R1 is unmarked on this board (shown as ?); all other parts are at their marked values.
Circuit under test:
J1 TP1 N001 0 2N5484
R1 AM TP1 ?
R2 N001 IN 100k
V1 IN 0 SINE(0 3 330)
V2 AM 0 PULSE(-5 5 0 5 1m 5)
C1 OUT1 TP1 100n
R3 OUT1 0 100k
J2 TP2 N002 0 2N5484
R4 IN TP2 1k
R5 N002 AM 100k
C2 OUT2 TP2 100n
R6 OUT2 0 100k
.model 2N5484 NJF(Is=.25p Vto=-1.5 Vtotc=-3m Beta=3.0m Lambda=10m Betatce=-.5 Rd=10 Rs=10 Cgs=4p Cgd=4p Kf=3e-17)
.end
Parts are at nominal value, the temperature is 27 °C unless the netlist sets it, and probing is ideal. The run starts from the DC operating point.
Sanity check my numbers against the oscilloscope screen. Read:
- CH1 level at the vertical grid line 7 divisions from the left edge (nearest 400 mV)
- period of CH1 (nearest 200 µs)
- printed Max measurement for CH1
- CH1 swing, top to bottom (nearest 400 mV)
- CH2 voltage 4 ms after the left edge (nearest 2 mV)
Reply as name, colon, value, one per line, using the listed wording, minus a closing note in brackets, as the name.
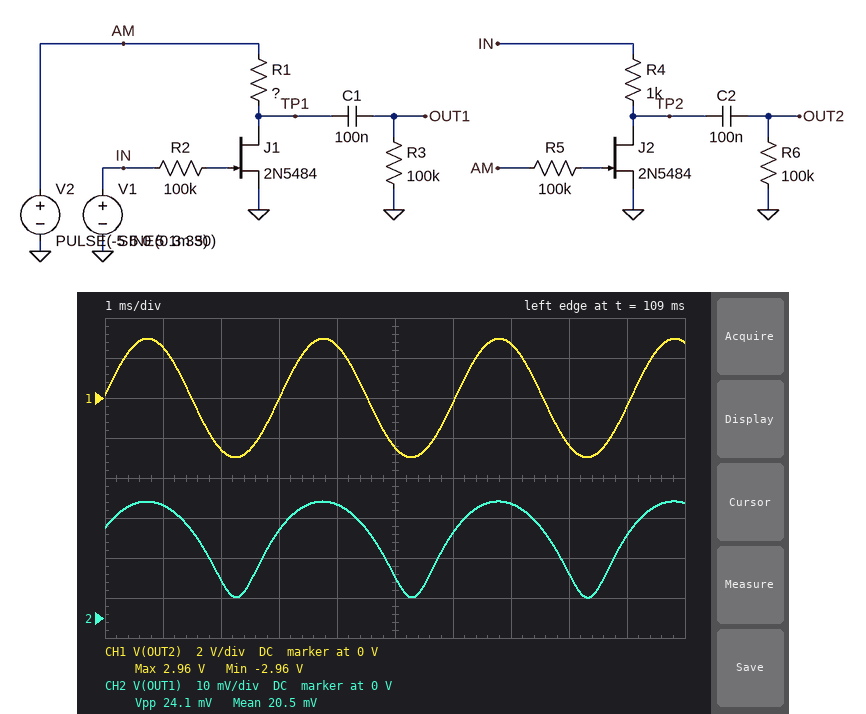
CH1 level at the vertical grid line 7 divisions from the left edge: 2.8 V
period of CH1: 3.0 ms
printed Max measurement for CH1: 2.96 V
CH1 swing, top to bottom: 6.0 V
CH2 voltage 4 ms after the left edge: 28 mV
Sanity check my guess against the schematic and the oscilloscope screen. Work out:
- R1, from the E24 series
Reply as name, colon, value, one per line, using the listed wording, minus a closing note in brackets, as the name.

R1, from the E24 series: 33 Ω
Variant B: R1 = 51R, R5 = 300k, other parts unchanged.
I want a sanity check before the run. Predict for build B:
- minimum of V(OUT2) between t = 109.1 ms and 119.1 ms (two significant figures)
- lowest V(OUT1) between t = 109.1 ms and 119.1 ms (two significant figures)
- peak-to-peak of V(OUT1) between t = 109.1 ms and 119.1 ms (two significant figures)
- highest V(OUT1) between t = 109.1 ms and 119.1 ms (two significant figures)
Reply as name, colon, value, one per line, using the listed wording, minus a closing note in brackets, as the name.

minimum of V(OUT2) between t = 109.1 ms and 119.1 ms: -3.0 V
lowest V(OUT1) between t = 109.1 ms and 119.1 ms: -5.9 mV
peak-to-peak of V(OUT1) between t = 109.1 ms and 119.1 ms: 41 mV
highest V(OUT1) between t = 109.1 ms and 119.1 ms: 35 mV
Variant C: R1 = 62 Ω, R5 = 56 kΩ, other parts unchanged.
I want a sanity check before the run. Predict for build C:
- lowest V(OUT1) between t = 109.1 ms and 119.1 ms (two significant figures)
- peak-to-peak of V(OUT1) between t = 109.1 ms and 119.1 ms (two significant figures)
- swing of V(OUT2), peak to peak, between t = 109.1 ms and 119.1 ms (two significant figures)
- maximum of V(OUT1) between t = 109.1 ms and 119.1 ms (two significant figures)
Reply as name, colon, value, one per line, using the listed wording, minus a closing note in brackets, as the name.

lowest V(OUT1) between t = 109.1 ms and 119.1 ms: -14 mV
peak-to-peak of V(OUT1) between t = 109.1 ms and 119.1 ms: 53 mV
swing of V(OUT2), peak to peak, between t = 109.1 ms and 119.1 ms: 5.9 V
maximum of V(OUT1) between t = 109.1 ms and 119.1 ms: 39 mV
